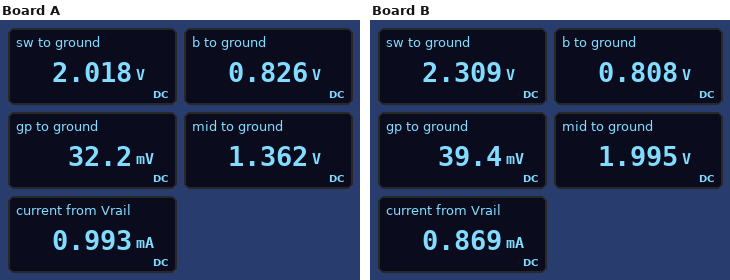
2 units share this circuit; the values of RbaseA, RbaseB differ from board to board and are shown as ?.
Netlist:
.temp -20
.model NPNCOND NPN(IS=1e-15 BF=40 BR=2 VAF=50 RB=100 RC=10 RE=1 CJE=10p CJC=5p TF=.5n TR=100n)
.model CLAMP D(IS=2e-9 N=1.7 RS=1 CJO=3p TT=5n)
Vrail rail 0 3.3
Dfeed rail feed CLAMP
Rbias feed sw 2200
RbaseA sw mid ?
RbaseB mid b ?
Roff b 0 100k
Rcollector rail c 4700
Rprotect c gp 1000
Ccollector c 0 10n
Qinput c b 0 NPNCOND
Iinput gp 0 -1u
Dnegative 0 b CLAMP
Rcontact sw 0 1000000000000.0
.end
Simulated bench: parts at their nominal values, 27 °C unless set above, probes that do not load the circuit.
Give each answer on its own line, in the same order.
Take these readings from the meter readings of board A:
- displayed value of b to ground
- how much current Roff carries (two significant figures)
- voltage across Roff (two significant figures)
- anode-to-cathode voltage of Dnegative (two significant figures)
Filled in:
0.826 V
8.3 µA
830 mV
-830 mV
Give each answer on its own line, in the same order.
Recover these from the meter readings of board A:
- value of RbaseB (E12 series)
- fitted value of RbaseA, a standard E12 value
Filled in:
1.8 kΩ
2.2 kΩ
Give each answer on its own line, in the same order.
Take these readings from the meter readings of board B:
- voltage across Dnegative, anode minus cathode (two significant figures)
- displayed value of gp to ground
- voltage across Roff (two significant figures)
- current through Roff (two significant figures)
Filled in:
-810 mV
39.4 mV
810 mV
8.1 µA
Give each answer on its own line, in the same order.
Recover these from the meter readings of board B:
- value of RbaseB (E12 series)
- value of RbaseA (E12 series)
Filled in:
6.8 kΩ
1.8 kΩ
